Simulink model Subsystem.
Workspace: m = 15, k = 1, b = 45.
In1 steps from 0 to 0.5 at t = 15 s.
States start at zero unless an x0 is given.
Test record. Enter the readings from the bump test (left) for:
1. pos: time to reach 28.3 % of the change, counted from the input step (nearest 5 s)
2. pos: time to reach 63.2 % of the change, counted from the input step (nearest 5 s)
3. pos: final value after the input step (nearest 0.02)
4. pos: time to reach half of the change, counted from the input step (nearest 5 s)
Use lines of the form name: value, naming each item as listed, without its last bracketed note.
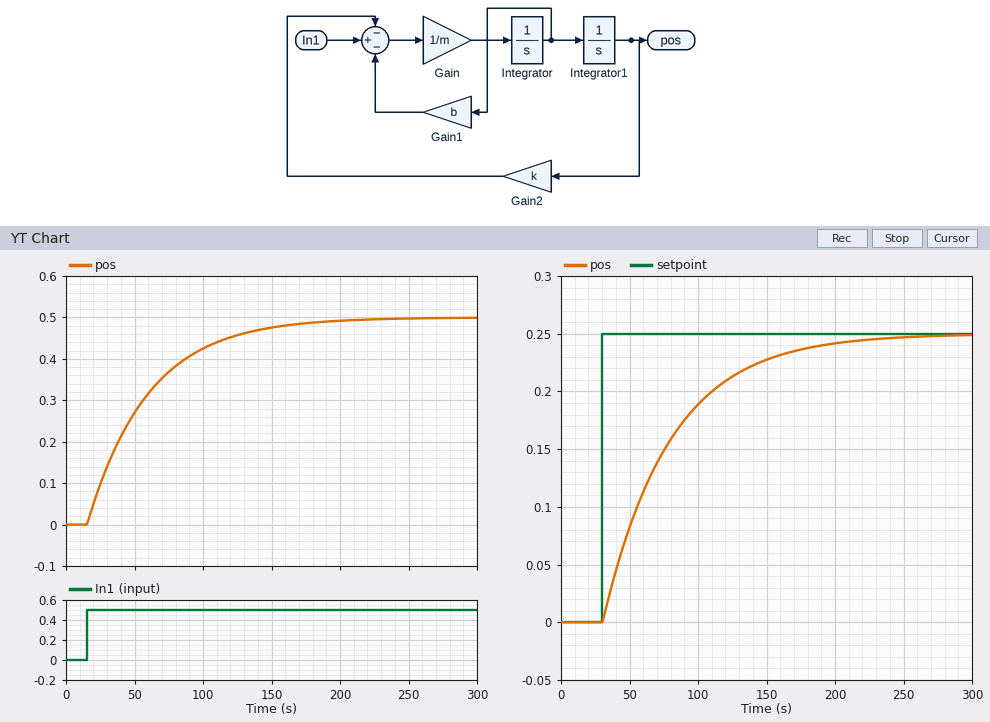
pos: time to reach 28.3 % of the change, counted from the input step: 15 s
pos: time to reach 63.2 % of the change, counted from the input step: 45 s
pos: final value after the input step: 0.50
pos: time to reach half of the change, counted from the input step: 30 s
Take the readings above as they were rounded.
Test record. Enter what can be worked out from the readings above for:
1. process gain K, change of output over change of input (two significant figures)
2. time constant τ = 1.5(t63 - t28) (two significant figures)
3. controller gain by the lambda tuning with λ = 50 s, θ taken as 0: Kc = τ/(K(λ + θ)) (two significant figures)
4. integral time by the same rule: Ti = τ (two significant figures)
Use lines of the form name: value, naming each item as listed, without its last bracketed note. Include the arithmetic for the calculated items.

process gain K, change of output over change of input: (0.5 - 0) / 0.5 = 1.0
time constant τ = 1.5(t63 - t28): 1.5 × (45 - 15) = 45 s
controller gain by the lambda tuning with λ = 50 s, θ taken as 0: Kc = τ/(K(λ + θ)): 45 / (1 × (50 + 0)) = 0.90
integral time by the same rule: Ti = τ: 45 s
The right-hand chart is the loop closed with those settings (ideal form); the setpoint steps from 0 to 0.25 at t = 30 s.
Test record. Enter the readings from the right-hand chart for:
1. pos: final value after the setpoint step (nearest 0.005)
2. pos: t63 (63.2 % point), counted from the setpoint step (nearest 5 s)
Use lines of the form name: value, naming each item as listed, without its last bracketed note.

pos: final value after the setpoint step: 0.250
pos: t63 (63.2 % point), counted from the setpoint step: 50 s
